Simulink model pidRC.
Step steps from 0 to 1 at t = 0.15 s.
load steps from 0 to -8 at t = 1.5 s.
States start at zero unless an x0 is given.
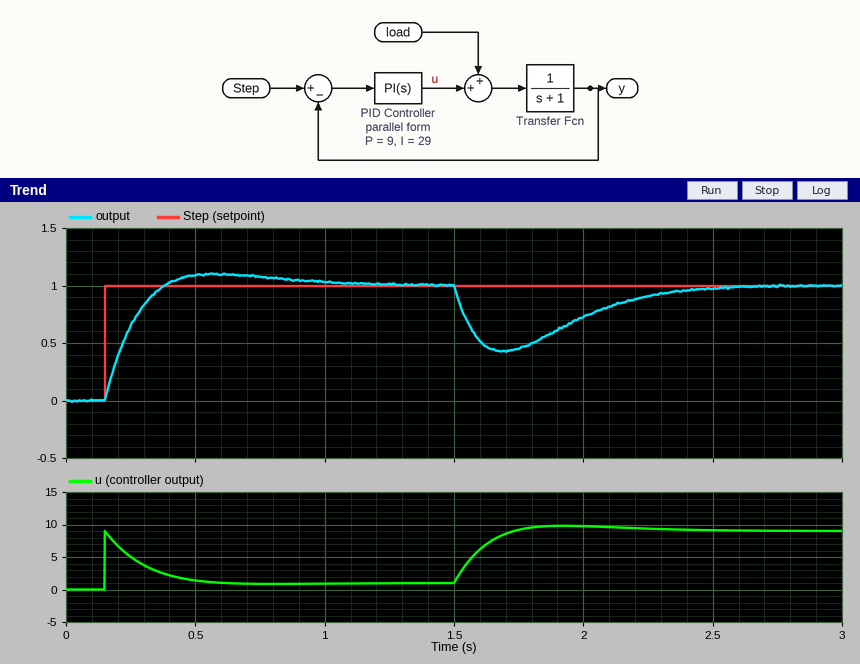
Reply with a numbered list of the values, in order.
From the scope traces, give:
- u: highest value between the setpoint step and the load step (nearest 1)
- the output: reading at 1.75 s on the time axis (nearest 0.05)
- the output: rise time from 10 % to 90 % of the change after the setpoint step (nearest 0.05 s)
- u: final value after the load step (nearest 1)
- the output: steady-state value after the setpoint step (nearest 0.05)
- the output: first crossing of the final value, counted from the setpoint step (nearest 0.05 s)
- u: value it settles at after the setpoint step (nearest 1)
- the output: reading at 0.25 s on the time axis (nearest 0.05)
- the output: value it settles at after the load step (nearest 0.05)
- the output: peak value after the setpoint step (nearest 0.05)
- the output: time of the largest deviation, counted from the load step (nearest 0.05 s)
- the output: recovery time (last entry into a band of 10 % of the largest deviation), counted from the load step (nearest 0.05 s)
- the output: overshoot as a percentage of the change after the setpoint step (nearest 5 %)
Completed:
1. 9
2. 0.45
3. 0.15 s
4. 9
5. 1.00
6. 0.25 s
7. 1
8. 0.65
9. 1.00
10. 1.10
11. 0.20 s
12. 0.85 s
13. 10 %
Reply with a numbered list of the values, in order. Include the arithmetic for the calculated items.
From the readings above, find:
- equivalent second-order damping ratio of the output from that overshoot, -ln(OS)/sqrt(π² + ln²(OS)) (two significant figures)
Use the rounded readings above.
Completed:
1. ln(0.1) = -2.303; 2.303 / sqrt(9.870 + 5.302) = 0.59
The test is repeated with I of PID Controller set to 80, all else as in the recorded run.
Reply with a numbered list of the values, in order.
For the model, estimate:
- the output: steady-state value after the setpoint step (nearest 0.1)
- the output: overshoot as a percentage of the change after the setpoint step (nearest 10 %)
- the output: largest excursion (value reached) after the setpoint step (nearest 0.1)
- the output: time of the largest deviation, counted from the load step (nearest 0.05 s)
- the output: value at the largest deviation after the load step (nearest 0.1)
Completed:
1. 1.0
2. 20 %
3. 1.2
4. 0.15 s
5. 0.5
